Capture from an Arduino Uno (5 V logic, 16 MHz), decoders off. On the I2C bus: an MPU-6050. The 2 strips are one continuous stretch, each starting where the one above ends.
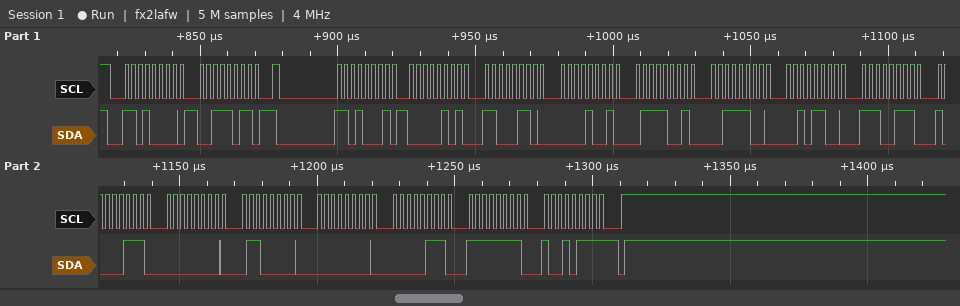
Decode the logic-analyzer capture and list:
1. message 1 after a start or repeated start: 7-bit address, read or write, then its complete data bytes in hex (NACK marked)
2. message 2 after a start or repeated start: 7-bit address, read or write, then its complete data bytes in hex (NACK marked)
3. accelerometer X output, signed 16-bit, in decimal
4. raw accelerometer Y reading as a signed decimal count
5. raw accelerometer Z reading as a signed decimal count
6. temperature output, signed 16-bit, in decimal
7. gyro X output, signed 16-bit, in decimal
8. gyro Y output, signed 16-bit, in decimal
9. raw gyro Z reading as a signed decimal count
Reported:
0x68 write: 3B
0x68 read: 05 C6 09 79 3C 2C E7 87 00 60 00 07 FF 97 NACK
1478
2425
15404
-6265
96
7
-105
